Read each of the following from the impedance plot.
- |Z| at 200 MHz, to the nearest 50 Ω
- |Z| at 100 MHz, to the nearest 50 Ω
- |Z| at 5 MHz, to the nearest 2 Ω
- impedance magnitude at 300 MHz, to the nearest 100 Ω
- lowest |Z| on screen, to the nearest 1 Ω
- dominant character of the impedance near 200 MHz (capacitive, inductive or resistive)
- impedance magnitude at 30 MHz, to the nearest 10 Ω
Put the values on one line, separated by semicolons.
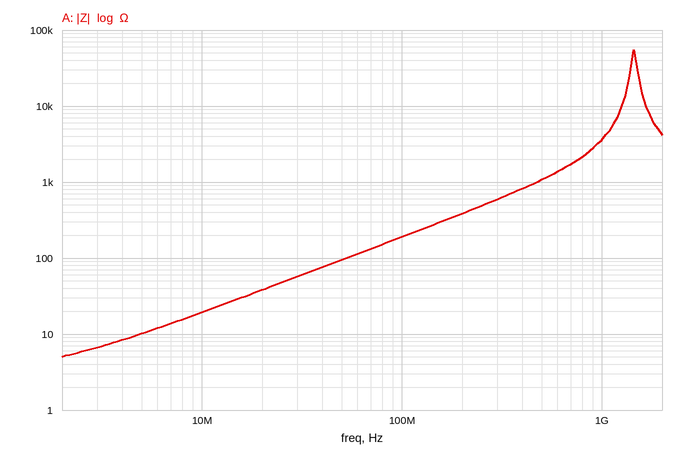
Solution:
400 Ω; 200 Ω; 10 Ω; 600 Ω; 5 Ω; inductive; 60 Ω
